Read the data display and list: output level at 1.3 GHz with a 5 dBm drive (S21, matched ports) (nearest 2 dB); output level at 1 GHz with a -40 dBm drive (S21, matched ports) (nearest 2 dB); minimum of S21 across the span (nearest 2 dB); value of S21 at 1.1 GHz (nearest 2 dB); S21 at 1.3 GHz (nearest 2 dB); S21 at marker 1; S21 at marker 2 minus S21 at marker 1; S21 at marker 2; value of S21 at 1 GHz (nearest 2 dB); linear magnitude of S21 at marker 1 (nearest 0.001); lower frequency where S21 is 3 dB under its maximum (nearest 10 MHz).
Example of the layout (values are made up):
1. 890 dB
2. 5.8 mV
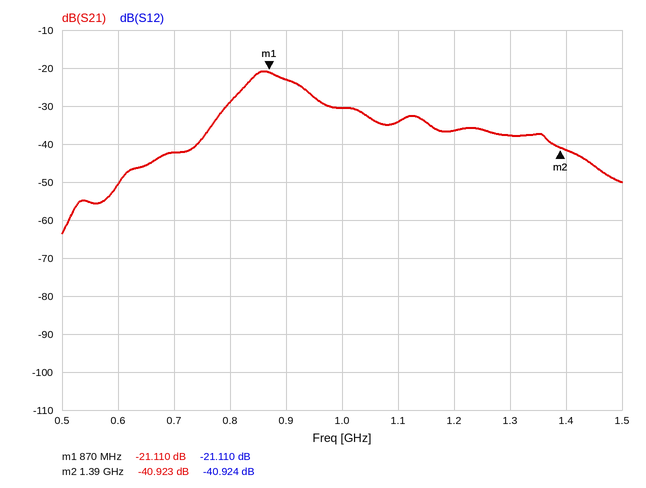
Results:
1. -32 dBm
2. -70 dBm
3. -64 dB
4. -34 dB
5. -38 dB
6. -21.110 dB
7. -19.813 dB
8. -40.923 dB
9. -30 dB
10. 0.088
11. 830 MHz
